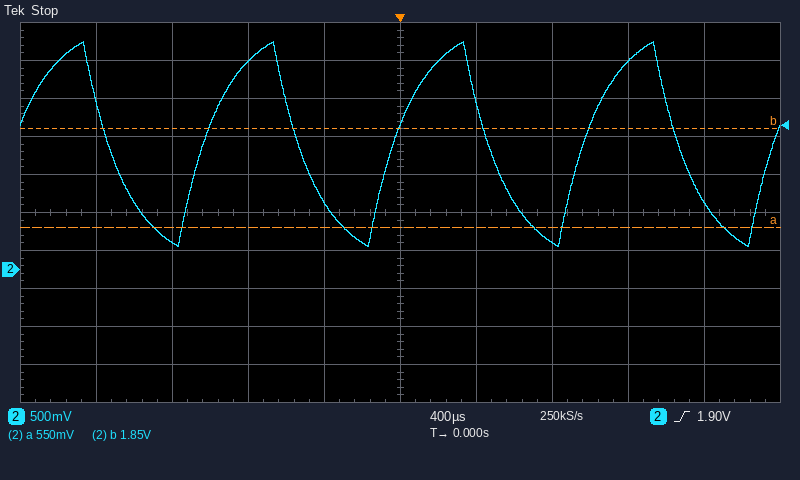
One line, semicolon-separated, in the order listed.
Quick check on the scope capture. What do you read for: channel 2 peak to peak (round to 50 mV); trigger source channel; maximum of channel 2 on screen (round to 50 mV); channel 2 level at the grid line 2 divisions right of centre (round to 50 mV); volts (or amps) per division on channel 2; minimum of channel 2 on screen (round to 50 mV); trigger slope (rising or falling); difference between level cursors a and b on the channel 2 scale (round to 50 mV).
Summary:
2.70 V; channel 2; 3.00 V; 350 mV; 500 mV; 300 mV; rising; 1.30 V
